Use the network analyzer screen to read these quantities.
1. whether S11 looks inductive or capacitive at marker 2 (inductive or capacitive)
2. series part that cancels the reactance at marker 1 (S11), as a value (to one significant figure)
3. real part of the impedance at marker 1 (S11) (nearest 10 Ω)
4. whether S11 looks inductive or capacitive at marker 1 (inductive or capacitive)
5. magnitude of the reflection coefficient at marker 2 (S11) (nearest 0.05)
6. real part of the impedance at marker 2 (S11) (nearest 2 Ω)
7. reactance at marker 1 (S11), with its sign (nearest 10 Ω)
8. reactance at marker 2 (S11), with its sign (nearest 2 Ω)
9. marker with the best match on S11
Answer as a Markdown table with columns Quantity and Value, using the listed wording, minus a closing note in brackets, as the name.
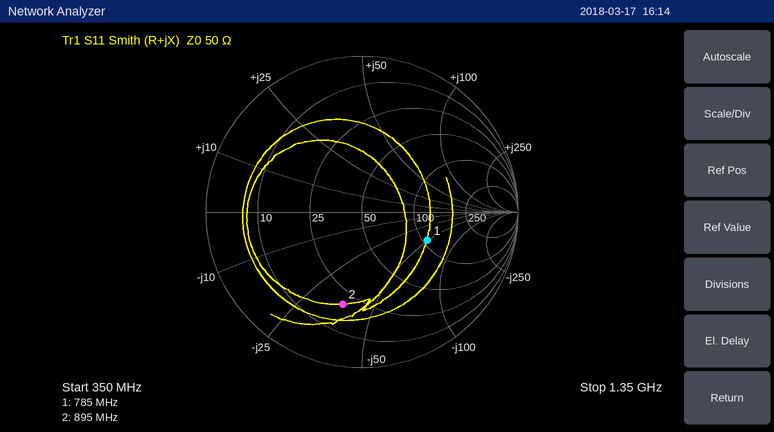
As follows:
| Quantity | Value |
|---|---|
| whether S11 looks inductive or capacitive at marker 2 | capacitive |
| series part that cancels the reactance at marker 1 (S11), as a value | 10 nH |
| real part of the impedance at marker 1 (S11) | 110 Ω |
| whether S11 looks inductive or capacitive at marker 1 | capacitive |
| magnitude of the reflection coefficient at marker 2 (S11) | 0.60 |
| real part of the impedance at marker 2 (S11) | 20 Ω |
| reactance at marker 1 (S11), with its sign | -50 Ω |
| reactance at marker 2 (S11), with its sign | -36 Ω |
| marker with the best match on S11 | marker 1 |
